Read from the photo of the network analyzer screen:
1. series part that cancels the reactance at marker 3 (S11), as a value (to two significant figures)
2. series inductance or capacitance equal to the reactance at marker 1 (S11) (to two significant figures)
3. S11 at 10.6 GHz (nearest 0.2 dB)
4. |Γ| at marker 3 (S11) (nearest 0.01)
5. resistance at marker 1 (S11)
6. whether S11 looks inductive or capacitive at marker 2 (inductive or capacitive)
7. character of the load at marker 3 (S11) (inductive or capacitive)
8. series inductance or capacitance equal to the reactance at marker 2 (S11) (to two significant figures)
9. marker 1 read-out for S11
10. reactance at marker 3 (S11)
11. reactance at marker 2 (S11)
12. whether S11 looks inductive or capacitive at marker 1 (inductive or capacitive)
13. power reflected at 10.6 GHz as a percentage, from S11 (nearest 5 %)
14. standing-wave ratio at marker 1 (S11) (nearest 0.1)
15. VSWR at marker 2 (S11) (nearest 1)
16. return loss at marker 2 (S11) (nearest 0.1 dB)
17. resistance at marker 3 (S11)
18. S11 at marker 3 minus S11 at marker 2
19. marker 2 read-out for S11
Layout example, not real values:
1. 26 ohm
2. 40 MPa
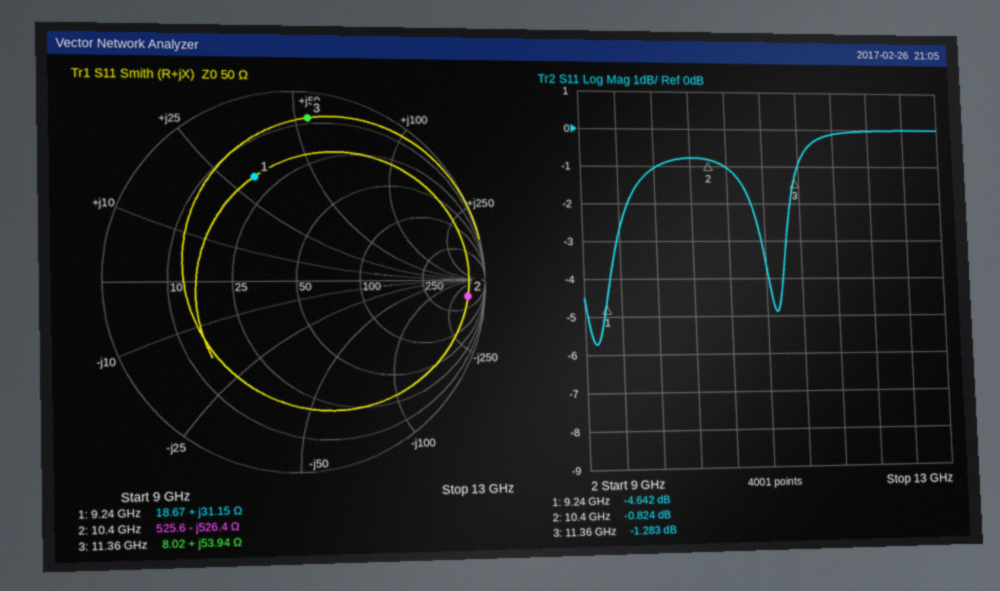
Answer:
1. 260 fF
2. 540 pH
3. -1.0 dB
4. 0.86
5. 18.67 Ω
6. capacitive
7. inductive
8. 29 fF
9. -4.642 dB
10. +53.94 Ω
11. -526.4 Ω
12. inductive
13. 80 %
14. 3.8
15. 21
16. 0.8 dB
17. 8.02 Ω
18. -0.459 dB
19. -0.824 dB
